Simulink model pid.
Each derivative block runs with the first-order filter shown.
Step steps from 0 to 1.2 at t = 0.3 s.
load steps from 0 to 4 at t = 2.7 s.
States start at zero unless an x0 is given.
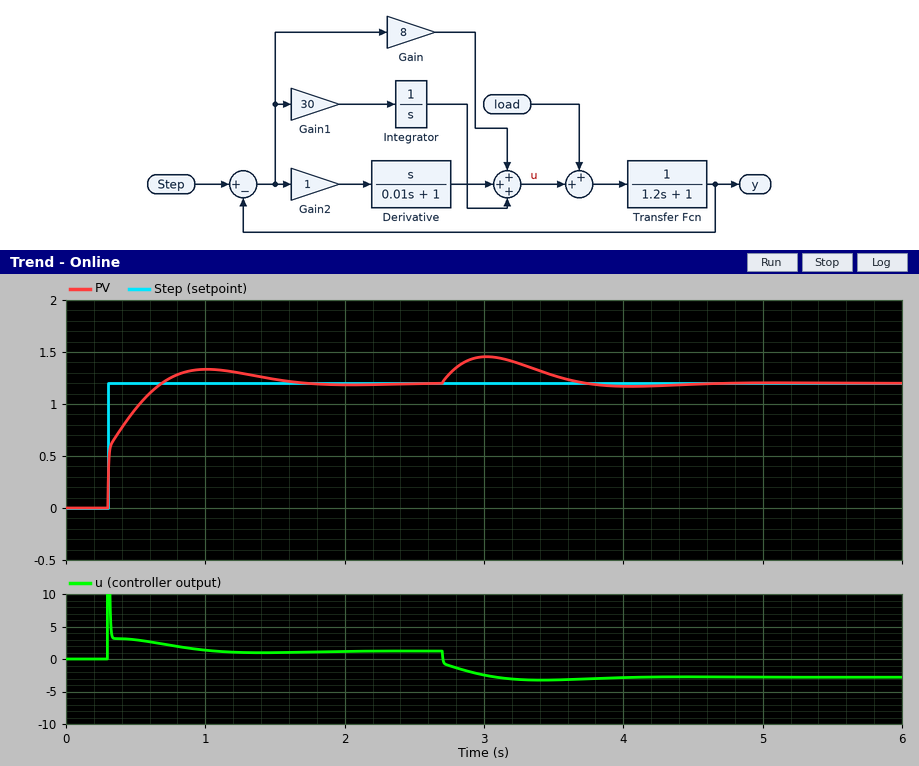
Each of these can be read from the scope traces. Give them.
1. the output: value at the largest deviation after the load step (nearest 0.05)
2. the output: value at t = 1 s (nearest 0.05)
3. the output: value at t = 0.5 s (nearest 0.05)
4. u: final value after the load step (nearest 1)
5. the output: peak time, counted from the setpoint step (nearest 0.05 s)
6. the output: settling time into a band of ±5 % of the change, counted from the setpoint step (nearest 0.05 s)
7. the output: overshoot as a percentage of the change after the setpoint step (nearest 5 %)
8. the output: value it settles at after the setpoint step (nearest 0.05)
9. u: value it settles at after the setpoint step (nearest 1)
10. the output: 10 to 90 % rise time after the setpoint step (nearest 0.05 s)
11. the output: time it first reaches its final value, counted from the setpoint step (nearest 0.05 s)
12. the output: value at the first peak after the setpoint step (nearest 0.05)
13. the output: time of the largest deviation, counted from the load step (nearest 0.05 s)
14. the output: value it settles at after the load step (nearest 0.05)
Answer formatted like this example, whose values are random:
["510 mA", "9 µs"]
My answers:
["1.45", "1.35", "0.95", "-3", "0.70 s", "1.10 s", "10 %", "1.20", "1", "0.30 s", "0.40 s", "1.35", "0.30 s", "1.20"]
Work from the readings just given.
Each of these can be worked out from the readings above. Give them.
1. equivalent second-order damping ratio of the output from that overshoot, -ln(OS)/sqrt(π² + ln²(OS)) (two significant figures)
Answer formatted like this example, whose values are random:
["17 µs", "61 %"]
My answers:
["0.59"]
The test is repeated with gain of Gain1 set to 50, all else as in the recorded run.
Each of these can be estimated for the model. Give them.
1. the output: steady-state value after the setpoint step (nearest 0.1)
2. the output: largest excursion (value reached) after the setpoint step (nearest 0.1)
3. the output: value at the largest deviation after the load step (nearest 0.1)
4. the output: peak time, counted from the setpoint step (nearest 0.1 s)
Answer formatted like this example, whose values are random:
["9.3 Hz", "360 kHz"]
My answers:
["1.2", "1.4", "1.4", "0.6 s"]
